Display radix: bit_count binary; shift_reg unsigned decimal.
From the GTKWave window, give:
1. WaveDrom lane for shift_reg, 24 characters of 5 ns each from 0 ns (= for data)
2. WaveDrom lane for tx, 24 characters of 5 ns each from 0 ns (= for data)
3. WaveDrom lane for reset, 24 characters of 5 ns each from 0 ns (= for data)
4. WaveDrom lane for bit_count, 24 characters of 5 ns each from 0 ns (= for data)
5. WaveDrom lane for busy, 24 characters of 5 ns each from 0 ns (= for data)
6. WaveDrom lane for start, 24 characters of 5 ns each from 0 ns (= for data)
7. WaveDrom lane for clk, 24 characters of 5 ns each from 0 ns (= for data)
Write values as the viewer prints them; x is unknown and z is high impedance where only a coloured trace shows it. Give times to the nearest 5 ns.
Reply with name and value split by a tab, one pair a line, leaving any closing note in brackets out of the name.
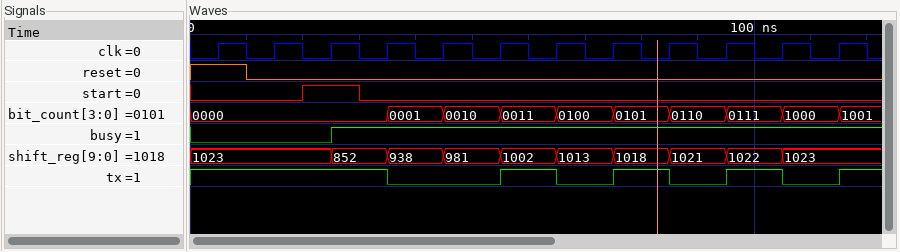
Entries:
WaveDrom lane for shift_reg, 24 characters of 5 ns each from 0 ns	{name: 'shift_reg', wave: '=....=.=.=.=.=.=.=.=.=..', data: '1023 852 938 981 1002 1013 1018 1021 1022 1023'}
WaveDrom lane for tx, 24 characters of 5 ns each from 0 ns	{name: 'tx', wave: '1......0...1.0.1.0.1.0.1'}
WaveDrom lane for reset, 24 characters of 5 ns each from 0 ns	{name: 'reset', wave: '1.0.....................'}
WaveDrom lane for bit_count, 24 characters of 5 ns each from 0 ns	{name: 'bit_count', wave: '=......=.=.=.=.=.=.=.=.=', data: '0000 0001 0010 0011 0100 0101 0110 0111 1000 1001'}
WaveDrom lane for busy, 24 characters of 5 ns each from 0 ns	{name: 'busy', wave: '0....1..................'}
WaveDrom lane for start, 24 characters of 5 ns each from 0 ns	{name: 'start', wave: '0...1.0.................'}
WaveDrom lane for clk, 24 characters of 5 ns each from 0 ns	{name: 'clk', wave: '010101010101010101010101'}
